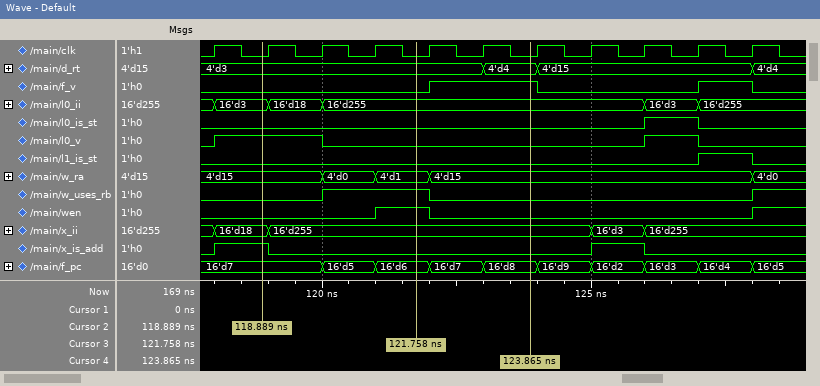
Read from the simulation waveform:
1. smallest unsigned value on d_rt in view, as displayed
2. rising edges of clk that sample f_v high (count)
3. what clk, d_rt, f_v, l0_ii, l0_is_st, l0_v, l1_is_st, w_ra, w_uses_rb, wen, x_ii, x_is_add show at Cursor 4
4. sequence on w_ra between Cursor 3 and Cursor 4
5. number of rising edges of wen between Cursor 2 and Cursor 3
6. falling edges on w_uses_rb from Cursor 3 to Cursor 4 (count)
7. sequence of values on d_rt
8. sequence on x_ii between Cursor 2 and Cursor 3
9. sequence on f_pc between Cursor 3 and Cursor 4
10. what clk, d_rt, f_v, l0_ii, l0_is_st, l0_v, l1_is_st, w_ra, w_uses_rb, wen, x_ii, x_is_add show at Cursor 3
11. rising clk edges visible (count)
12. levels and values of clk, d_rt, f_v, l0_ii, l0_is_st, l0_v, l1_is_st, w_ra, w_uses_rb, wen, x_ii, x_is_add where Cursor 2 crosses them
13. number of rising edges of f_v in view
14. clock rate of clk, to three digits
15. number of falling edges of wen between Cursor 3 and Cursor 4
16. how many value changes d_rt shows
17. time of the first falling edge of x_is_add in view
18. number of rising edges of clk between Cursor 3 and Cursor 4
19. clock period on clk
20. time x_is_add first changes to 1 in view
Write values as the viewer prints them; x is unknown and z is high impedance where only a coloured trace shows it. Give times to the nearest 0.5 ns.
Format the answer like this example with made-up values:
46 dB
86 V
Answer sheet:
4'd3
3
clk=0, d_rt=4'd4, f_v=1, l0_ii=16'd255, l0_is_st=0, l0_v=0, l1_is_st=0, w_ra=4'd15, w_uses_rb=0, wen=0, x_ii=16'd255, x_is_add=0
4'd1, 4'd15
1
1
4'd3, 4'd4, 4'd15, 4'd4
16'd18, 16'd255
16'd6, 16'd7, 16'd8
clk=0, d_rt=4'd3, f_v=0, l0_ii=16'd255, l0_is_st=0, l0_v=0, l1_is_st=0, w_ra=4'd1, w_uses_rb=1, wen=1, x_ii=16'd255, x_is_add=0
11
clk=0, d_rt=4'd3, f_v=0, l0_ii=16'd3, l0_is_st=0, l0_v=1, l1_is_st=0, w_ra=4'd15, w_uses_rb=0, wen=0, x_ii=16'd18, x_is_add=1
2
1.00 GHz
1
3
119 ns
2
1 ns
118 ns
